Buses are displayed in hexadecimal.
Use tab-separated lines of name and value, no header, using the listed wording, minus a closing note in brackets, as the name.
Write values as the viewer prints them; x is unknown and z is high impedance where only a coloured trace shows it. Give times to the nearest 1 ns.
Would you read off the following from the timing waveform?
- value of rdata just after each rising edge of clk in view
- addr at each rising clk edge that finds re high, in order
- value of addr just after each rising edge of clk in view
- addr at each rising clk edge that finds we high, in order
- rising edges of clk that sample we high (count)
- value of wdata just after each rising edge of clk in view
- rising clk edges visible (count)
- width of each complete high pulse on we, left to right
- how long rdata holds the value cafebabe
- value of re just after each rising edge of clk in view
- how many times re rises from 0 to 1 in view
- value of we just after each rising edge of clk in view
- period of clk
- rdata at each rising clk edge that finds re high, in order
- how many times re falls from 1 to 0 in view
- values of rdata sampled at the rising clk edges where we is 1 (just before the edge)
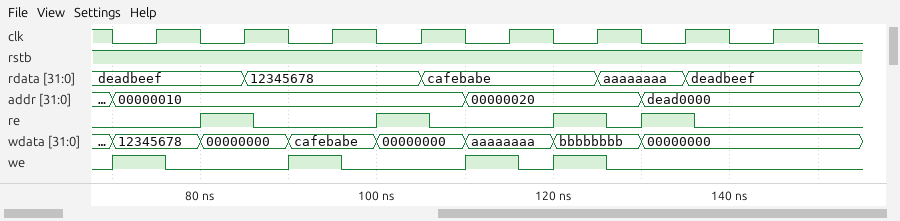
value of rdata just after each rising edge of clk in view	deadbeef, 12345678, 12345678, cafebabe, cafebabe, aaaaaaaa, deadbeef, deadbeef
addr at each rising clk edge that finds re high, in order	00000010, 00000010, 00000020, dead0000
value of addr just after each rising edge of clk in view	00000010, 00000010, 00000010, 00000010, 00000020, 00000020, dead0000, dead0000
addr at each rising clk edge that finds we high, in order	00000010, 00000010, 00000020, 00000020
rising edges of clk that sample we high	4
value of wdata just after each rising edge of clk in view	12345678, 00000000, cafebabe, 00000000, aaaaaaaa, bbbbbbbb, 00000000, 00000000
rising clk edges visible	8
width of each complete high pulse on we, left to right	6 ns, 6 ns, 6 ns, 6 ns
how long rdata holds the value cafebabe	20 ns
value of re just after each rising edge of clk in view	0 1 0 1 0 1 1 0
how many times re rises from 0 to 1 in view	4
value of we just after each rising edge of clk in view	1 0 1 0 1 1 0 0
period of clk	10 ns
rdata at each rising clk edge that finds re high, in order	deadbeef, 12345678, cafebabe, aaaaaaaa
how many times re falls from 1 to 0 in view	4
values of rdata sampled at the rising clk edges where we is 1	deadbeef, 12345678, cafebabe, cafebabe
